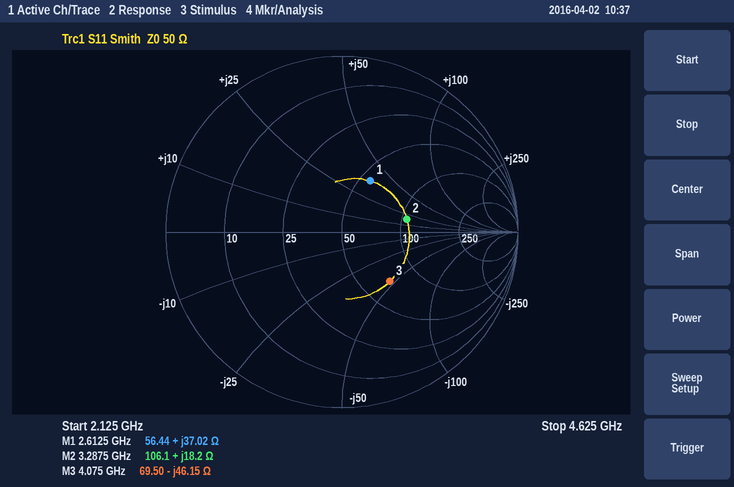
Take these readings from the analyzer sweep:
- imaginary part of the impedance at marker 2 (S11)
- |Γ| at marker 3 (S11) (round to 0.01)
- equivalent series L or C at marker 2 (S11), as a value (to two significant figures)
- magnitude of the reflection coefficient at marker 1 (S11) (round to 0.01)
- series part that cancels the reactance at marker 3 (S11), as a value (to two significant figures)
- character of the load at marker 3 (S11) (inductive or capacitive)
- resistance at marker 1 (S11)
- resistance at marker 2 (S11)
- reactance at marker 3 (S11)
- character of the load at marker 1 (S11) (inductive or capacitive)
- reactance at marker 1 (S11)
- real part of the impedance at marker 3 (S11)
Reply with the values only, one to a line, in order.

+18.2 Ω
0.39
880 pH
0.33
1.8 nH
capacitive
56.44 Ω
106.1 Ω
-46.15 Ω
inductive
+37.02 Ω
69.50 Ω
